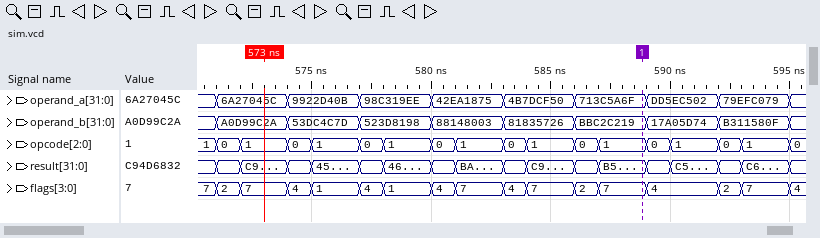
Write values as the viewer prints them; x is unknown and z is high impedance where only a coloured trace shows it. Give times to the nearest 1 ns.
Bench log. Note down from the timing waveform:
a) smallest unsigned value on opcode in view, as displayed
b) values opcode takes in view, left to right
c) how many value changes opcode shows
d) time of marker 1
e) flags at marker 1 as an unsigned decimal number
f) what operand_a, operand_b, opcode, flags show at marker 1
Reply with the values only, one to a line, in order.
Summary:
0
1, 0, 1, 0, 1, 0, 1, 0, 1, 0, 1, 0, 1, 0, 1, 0, 1, 0
17
589 ns
7
operand_a=713C5A6F, operand_b=BBC2C219, opcode=1, flags=7
